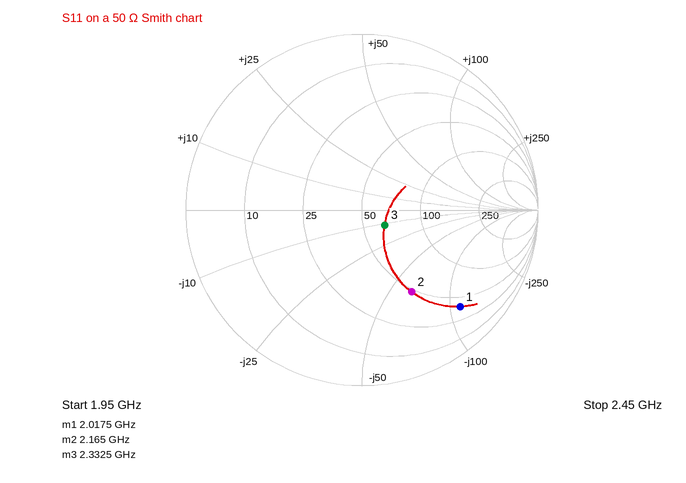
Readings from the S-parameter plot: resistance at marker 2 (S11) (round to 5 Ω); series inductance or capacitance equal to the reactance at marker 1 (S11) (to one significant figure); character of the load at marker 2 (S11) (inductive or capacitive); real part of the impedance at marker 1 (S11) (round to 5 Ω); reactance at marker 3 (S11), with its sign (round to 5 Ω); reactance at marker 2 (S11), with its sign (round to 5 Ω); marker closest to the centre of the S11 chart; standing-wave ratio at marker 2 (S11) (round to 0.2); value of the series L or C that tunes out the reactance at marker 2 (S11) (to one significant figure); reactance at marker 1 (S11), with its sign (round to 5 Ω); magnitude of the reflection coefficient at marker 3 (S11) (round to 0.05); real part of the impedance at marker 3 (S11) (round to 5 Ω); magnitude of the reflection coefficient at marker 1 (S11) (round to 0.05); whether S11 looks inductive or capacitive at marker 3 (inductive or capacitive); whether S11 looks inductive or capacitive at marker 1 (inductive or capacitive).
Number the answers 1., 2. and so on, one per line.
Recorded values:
1. 50 Ω
2. 700 fF
3. capacitive
4. 40 Ω
5. -10 Ω
6. -65 Ω
7. marker 3
8. 3.4
9. 5 nH
10. -110 Ω
11. 0.15
12. 65 Ω
13. 0.80
14. capacitive
15. capacitive
